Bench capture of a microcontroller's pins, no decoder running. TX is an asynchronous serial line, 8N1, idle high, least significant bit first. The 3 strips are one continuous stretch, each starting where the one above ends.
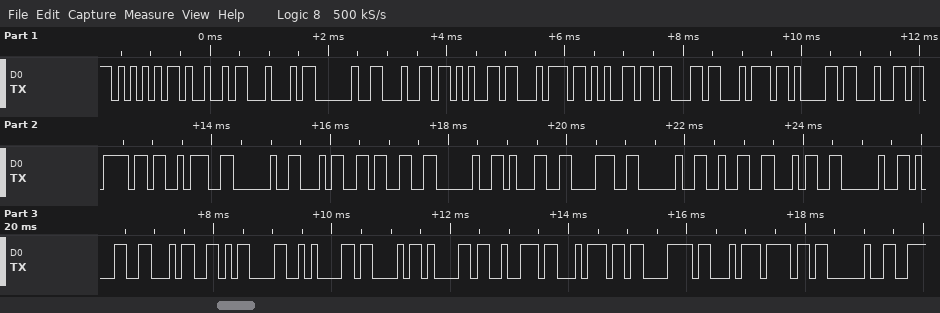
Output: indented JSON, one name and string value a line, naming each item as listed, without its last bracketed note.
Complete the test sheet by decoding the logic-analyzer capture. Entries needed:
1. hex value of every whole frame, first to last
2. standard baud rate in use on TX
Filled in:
{
  "hex value of every whole frame, first to last": "0x55 0x49 0x44 0x20 0x64 0x65 0x74 0x65 0x63 0x74 0x61 0x64 0x6F 0x3A 0x20 0x34 0x33 0x20 0x31 0x38 0x20 0x32 0x34 0x20 0x31 0x34 0x0D 0x0A 0x43 0x61 0x72 0x74 0xC3 0xA3 0x6F 0x20",
  "standard baud rate in use on TX": "9600 baud"
}
